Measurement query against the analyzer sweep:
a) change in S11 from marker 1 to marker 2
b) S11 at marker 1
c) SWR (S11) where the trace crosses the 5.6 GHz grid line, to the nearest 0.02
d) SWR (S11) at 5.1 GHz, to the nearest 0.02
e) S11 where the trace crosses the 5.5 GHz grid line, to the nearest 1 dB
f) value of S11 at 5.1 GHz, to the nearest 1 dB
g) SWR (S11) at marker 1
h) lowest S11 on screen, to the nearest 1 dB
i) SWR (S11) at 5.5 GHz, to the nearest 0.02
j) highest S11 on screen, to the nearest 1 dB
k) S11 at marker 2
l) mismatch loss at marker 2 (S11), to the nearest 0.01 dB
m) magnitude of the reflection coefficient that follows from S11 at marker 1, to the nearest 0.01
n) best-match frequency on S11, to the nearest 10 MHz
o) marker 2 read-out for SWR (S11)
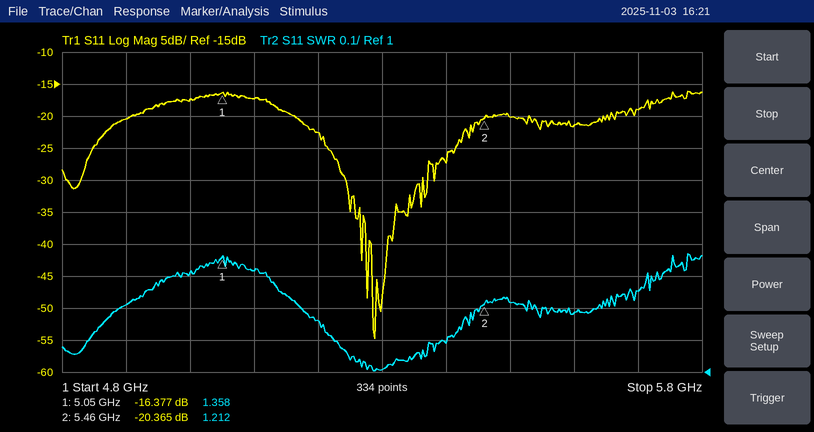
-3.988 dB
-16.377 dB
1.18
1.32
-20 dB
-17 dB
1.358
-55 dB
1.22
-16 dB
-20.365 dB
0.04 dB
0.15
5.29 GHz
1.212
